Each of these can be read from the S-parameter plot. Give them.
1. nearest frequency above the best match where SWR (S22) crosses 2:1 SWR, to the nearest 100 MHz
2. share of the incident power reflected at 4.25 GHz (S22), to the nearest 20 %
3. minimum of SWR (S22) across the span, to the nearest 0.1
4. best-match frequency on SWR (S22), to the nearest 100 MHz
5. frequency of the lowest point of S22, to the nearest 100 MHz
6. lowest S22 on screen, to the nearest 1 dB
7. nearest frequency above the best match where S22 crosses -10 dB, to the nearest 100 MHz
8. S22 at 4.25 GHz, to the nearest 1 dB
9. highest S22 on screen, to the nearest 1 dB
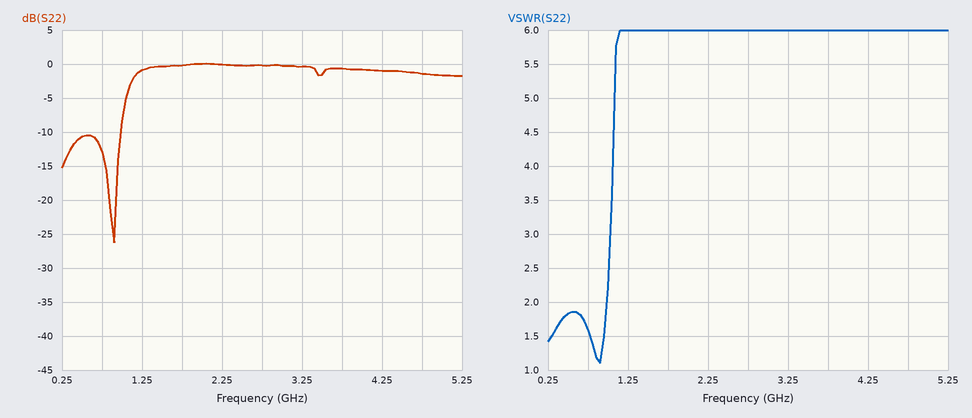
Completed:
1.0 GHz
80 %
1.1
900 MHz
900 MHz
-26 dB
1.0 GHz
-1 dB
0 dB
